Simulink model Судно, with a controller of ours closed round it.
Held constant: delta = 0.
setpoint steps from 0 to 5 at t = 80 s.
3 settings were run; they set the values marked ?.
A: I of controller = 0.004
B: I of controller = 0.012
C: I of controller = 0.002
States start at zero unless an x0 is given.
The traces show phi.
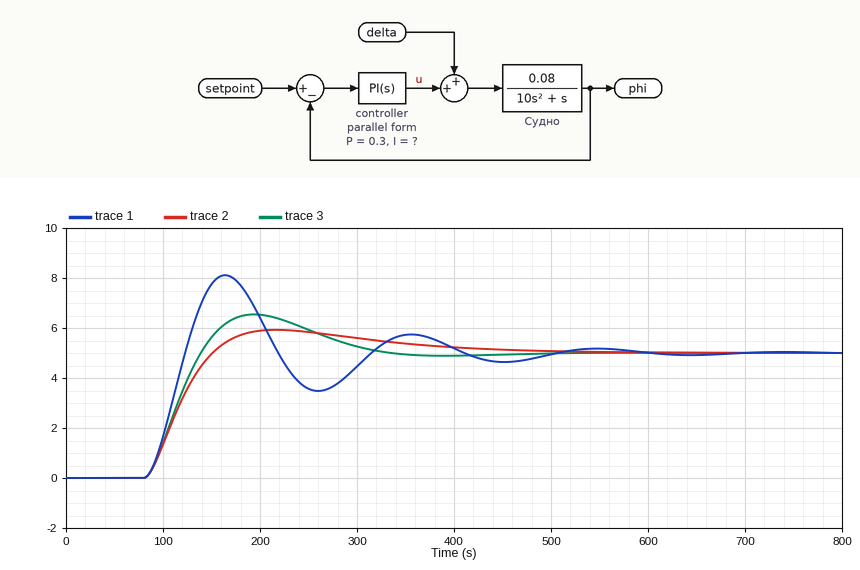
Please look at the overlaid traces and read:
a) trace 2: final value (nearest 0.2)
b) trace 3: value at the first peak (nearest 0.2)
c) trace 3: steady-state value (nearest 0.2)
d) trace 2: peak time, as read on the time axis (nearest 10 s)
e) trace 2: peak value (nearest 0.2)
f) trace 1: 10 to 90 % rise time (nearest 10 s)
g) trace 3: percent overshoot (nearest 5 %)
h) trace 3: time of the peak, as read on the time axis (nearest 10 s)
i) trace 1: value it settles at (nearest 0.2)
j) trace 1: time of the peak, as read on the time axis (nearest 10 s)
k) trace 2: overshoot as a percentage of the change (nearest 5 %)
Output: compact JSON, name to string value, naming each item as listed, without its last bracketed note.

{"trace 2: final value": "5.0", "trace 3: value at the first peak": "6.6", "trace 3: steady-state value": "5.0", "trace 2: peak time, as read on the time axis": "220 s", "trace 2: peak value": "6.0", "trace 1: 10 to 90 % rise time": "30 s", "trace 3: percent overshoot": "30 %", "trace 3: time of the peak, as read on the time axis": "190 s", "trace 1: value it settles at": "5.0", "trace 1: time of the peak, as read on the time axis": "160 s", "trace 2: overshoot as a percentage of the change": "20 %"}
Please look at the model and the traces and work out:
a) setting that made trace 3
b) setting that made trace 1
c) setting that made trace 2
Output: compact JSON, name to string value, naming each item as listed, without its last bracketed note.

{"setting that made trace 3": "A", "setting that made trace 1": "B", "setting that made trace 2": "C"}
